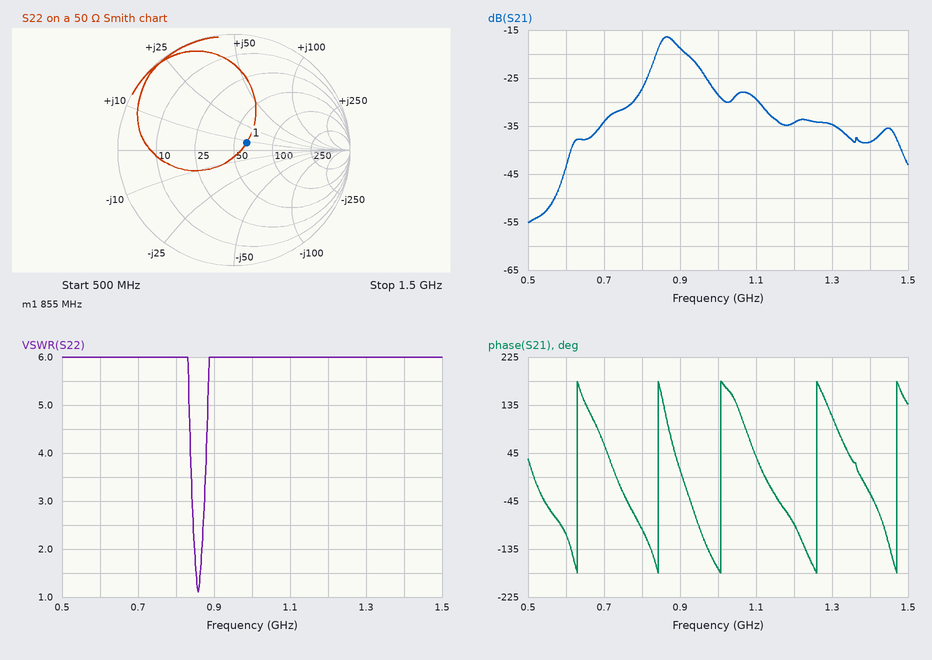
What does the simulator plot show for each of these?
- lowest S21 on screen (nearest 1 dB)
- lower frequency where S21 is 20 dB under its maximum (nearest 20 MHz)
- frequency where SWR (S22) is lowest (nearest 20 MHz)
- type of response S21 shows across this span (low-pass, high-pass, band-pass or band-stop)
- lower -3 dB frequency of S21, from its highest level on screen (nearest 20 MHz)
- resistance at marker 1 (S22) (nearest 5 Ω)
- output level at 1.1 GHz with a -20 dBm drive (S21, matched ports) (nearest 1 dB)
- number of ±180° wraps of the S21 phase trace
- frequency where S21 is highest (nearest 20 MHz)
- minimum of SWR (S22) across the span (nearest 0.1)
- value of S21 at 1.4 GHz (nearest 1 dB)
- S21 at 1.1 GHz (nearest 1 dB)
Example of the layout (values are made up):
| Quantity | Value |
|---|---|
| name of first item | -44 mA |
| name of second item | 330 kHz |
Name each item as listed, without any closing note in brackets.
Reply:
| Quantity | Value |
|---|---|
| lowest S21 on screen | -55 dB |
| lower frequency where S21 is 20 dB under its maximum | 680 MHz |
| frequency where SWR (S22) is lowest | 860 MHz |
| type of response S21 shows across this span | band-pass |
| lower -3 dB frequency of S21, from its highest level on screen | 840 MHz |
| resistance at marker 1 (S22) | 60 Ω |
| output level at 1.1 GHz with a -20 dBm drive (S21, matched ports) | -49 dBm |
| number of ±180° wraps of the S21 phase trace | 5 |
| frequency where S21 is highest | 860 MHz |
| minimum of SWR (S22) across the span | 1.1 |
| value of S21 at 1.4 GHz | -38 dB |
| S21 at 1.1 GHz | -29 dB |
